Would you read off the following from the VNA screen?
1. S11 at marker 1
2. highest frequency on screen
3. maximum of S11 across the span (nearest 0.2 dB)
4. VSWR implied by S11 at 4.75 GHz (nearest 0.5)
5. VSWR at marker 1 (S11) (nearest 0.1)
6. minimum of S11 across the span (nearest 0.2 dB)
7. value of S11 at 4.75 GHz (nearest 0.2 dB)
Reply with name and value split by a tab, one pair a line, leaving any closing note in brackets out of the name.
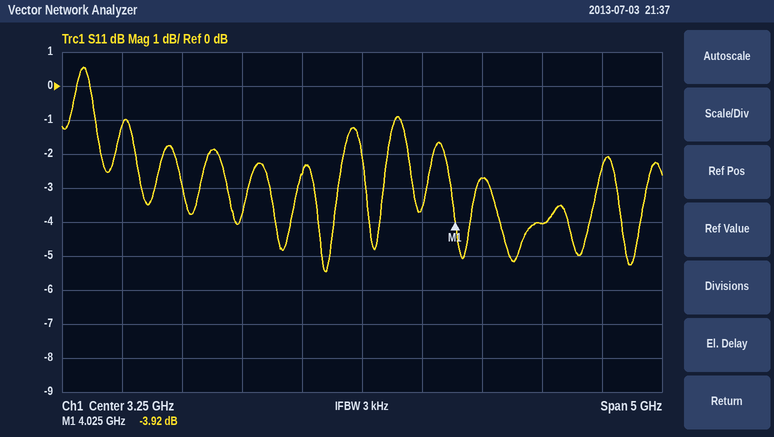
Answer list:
S11 at marker 1	-3.92 dB
highest frequency on screen	5.75 GHz
maximum of S11 across the span	0.6 dB
VSWR implied by S11 at 4.75 GHz	4.5
VSWR at marker 1 (S11)	4.5
minimum of S11 across the span	-5.4 dB
value of S11 at 4.75 GHz	-4.0 dB
